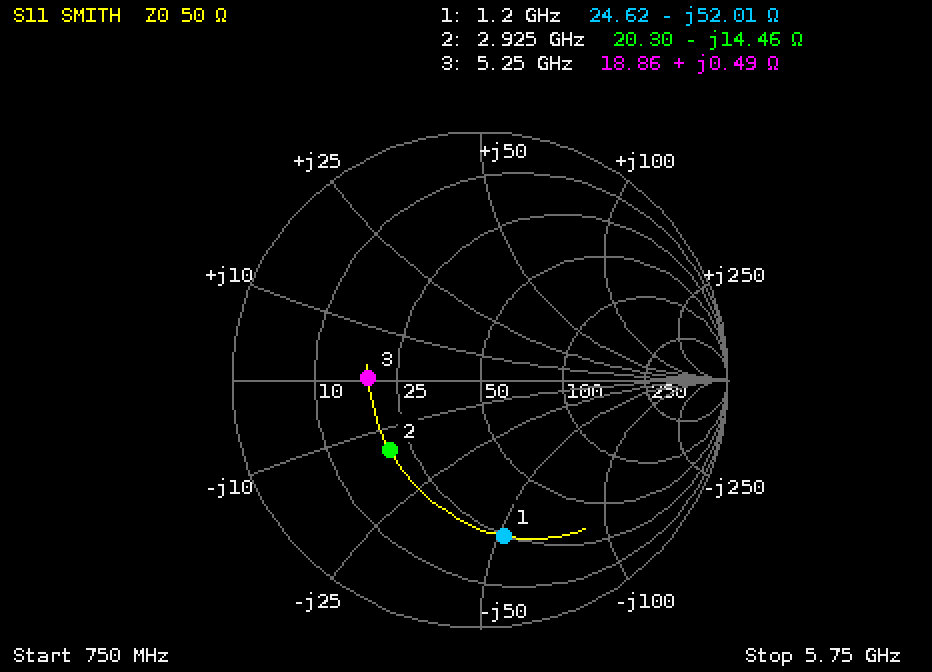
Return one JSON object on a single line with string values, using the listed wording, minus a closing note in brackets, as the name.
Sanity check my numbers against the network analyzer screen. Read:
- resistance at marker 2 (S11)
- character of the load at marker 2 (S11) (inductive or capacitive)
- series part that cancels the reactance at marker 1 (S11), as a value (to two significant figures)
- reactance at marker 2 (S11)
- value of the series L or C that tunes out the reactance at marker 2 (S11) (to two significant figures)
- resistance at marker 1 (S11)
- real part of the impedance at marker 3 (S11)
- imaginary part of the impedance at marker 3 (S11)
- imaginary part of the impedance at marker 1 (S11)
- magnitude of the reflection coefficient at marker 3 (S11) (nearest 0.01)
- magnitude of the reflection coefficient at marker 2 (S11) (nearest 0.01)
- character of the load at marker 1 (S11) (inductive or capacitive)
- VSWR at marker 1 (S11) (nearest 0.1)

{"resistance at marker 2": "20.30 Ω", "character of the load at marker 2 (S11)": "capacitive", "series part that cancels the reactance at marker 1 (S11), as a value": "6.9 nH", "reactance at marker 2": "-14.46 Ω", "value of the series L or C that tunes out the reactance at marker 2 (S11)": "790 pH", "resistance at marker 1": "24.62 Ω", "real part of the impedance at marker 3": "18.86 Ω", "imaginary part of the impedance at marker 3": "+0.49 Ω", "imaginary part of the impedance at marker 1": "-52.01 Ω", "magnitude of the reflection coefficient at marker 3 (S11)": "0.45", "magnitude of the reflection coefficient at marker 2 (S11)": "0.46", "character of the load at marker 1 (S11)": "capacitive", "VSWR at marker 1 (S11)": "4.5"}
